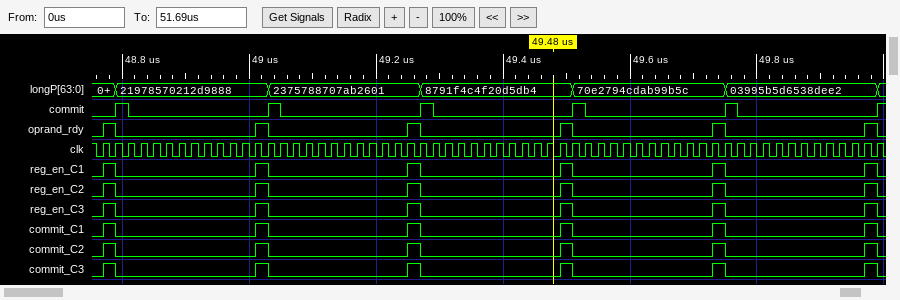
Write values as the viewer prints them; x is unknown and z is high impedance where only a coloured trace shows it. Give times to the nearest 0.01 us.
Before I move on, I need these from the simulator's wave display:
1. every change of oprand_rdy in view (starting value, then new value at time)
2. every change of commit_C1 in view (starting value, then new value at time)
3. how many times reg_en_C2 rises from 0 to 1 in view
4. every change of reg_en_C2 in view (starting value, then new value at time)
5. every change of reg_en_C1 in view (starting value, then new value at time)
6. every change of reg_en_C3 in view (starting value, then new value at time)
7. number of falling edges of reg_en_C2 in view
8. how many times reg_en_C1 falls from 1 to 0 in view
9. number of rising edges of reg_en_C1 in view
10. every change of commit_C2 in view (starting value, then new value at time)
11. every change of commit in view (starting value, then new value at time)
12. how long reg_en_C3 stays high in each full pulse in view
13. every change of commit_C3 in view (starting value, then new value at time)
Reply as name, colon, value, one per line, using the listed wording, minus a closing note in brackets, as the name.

every change of oprand_rdy in view: 0, 1 at 48.77 us, 0 at 48.79 us, 1 at 49.01 us, 0 at 49.03 us, 1 at 49.25 us, 0 at 49.27 us, 1 at 49.49 us, 0 at 49.51 us, 1 at 49.73 us, 0 at 49.75 us, 1 at 49.97 us, 0 at 49.99 us
every change of commit_C1 in view: 0, 1 at 48.77 us, 0 at 48.79 us, 1 at 49.01 us, 0 at 49.03 us, 1 at 49.25 us, 0 at 49.27 us, 1 at 49.49 us, 0 at 49.51 us, 1 at 49.73 us, 0 at 49.75 us, 1 at 49.97 us, 0 at 49.99 us
how many times reg_en_C2 rises from 0 to 1 in view: 6
every change of reg_en_C2 in view: 0, 1 at 48.77 us, 0 at 48.79 us, 1 at 49.01 us, 0 at 49.03 us, 1 at 49.25 us, 0 at 49.27 us, 1 at 49.49 us, 0 at 49.51 us, 1 at 49.73 us, 0 at 49.75 us, 1 at 49.97 us, 0 at 49.99 us
every change of reg_en_C1 in view: 0, 1 at 48.77 us, 0 at 48.79 us, 1 at 49.01 us, 0 at 49.03 us, 1 at 49.25 us, 0 at 49.27 us, 1 at 49.49 us, 0 at 49.51 us, 1 at 49.73 us, 0 at 49.75 us, 1 at 49.97 us, 0 at 49.99 us
every change of reg_en_C3 in view: 0, 1 at 48.77 us, 0 at 48.79 us, 1 at 49.01 us, 0 at 49.03 us, 1 at 49.25 us, 0 at 49.27 us, 1 at 49.49 us, 0 at 49.51 us, 1 at 49.73 us, 0 at 49.75 us, 1 at 49.97 us, 0 at 49.99 us
number of falling edges of reg_en_C2 in view: 6
how many times reg_en_C1 falls from 1 to 0 in view: 6
number of rising edges of reg_en_C1 in view: 6
every change of commit_C2 in view: 0, 1 at 48.77 us, 0 at 48.79 us, 1 at 49.01 us, 0 at 49.03 us, 1 at 49.25 us, 0 at 49.27 us, 1 at 49.49 us, 0 at 49.51 us, 1 at 49.73 us, 0 at 49.75 us, 1 at 49.97 us, 0 at 49.99 us
every change of commit in view: 0, 1 at 48.79 us, 0 at 48.81 us, 1 at 49.03 us, 0 at 49.05 us, 1 at 49.27 us, 0 at 49.29 us, 1 at 49.51 us, 0 at 49.53 us, 1 at 49.75 us, 0 at 49.77 us, 1 at 49.99 us
how long reg_en_C3 stays high in each full pulse in view: 0.02 us, 0.02 us, 0.02 us, 0.02 us, 0.02 us, 0.02 us
every change of commit_C3 in view: 0, 1 at 48.77 us, 0 at 48.79 us, 1 at 49.01 us, 0 at 49.03 us, 1 at 49.25 us, 0 at 49.27 us, 1 at 49.49 us, 0 at 49.51 us, 1 at 49.73 us, 0 at 49.75 us, 1 at 49.97 us, 0 at 49.99 us
